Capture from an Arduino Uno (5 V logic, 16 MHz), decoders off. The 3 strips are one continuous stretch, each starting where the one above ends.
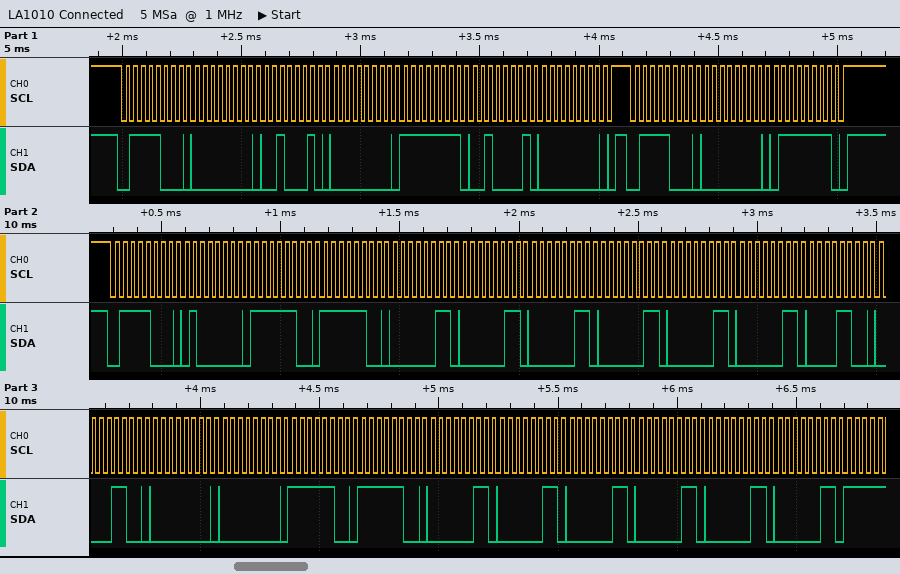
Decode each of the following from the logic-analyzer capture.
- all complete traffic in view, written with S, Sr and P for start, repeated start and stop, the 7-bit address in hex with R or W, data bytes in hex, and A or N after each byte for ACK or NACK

S 3CW A 00 A 22 A 00 A FF A 21 A 00 A P S 3CW A 00 A 7F A P S 3CW A 40 A FC A FC A 03 A 03 A 03 A 03 A 03 A 03 A 0C A 0C A 00 A 00 A FC A FC A 03 A 03 A 03 A 03 A 03 A 03 A
